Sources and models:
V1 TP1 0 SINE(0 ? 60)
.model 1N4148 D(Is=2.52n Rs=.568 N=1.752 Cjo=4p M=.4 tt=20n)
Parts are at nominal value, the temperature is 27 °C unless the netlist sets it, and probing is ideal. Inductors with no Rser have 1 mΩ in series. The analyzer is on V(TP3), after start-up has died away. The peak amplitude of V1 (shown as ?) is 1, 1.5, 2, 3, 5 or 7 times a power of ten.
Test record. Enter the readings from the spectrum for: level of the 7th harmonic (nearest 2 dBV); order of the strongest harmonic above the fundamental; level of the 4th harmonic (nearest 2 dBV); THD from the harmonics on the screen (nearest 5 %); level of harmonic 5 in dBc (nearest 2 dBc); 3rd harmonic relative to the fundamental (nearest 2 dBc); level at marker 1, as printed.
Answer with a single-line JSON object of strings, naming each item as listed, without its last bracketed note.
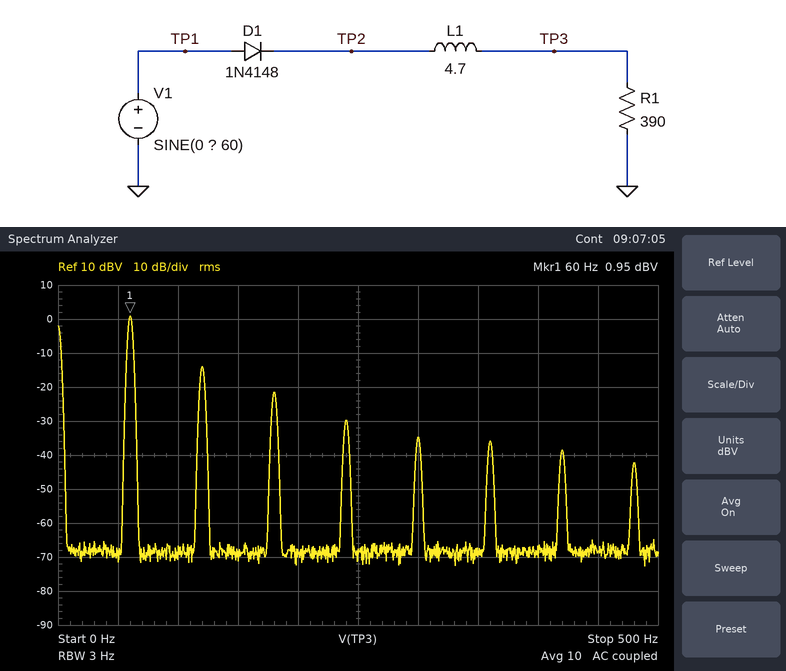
{"level of the 7th harmonic": "-38 dBV", "order of the strongest harmonic above the fundamental": "2", "level of the 4th harmonic": "-30 dBV", "THD from the harmonics on the screen": "20 %", "level of harmonic 5 in dBc": "-36 dBc", "3rd harmonic relative to the fundamental": "-22 dBc", "level at marker 1, as printed": "0.95 dBV"}
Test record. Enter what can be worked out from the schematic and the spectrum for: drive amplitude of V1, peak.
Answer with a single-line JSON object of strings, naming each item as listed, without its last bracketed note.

{"drive amplitude of V1, peak": "10 V"}
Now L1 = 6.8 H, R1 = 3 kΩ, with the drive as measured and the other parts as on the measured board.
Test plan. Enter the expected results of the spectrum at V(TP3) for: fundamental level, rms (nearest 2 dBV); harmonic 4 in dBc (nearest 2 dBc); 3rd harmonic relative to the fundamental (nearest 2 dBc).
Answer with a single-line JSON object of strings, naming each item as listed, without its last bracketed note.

{"fundamental level, rms": "8 dBV", "harmonic 4 in dBc": "-26 dBc", "3rd harmonic relative to the fundamental": "-26 dBc"}
